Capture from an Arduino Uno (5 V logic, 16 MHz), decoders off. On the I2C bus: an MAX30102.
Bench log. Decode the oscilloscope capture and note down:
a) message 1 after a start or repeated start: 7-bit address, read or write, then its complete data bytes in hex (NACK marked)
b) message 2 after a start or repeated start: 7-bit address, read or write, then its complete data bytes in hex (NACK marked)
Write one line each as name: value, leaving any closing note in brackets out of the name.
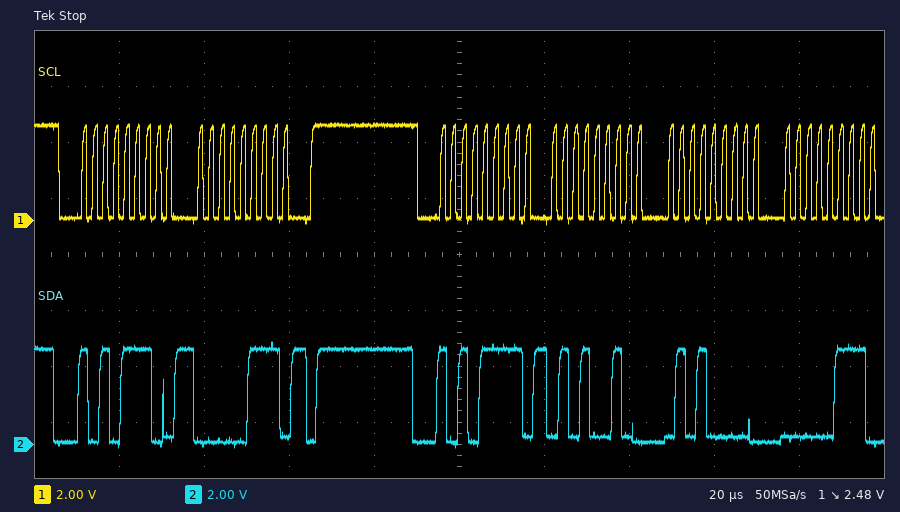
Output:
message 1 after a start or repeated start: 7-bit address, read or write, then its complete data bytes in hex: 0x57 write: 07
message 2 after a start or repeated start: 7-bit address, read or write, then its complete data bytes in hex: 0x57 read: 52 50 07
